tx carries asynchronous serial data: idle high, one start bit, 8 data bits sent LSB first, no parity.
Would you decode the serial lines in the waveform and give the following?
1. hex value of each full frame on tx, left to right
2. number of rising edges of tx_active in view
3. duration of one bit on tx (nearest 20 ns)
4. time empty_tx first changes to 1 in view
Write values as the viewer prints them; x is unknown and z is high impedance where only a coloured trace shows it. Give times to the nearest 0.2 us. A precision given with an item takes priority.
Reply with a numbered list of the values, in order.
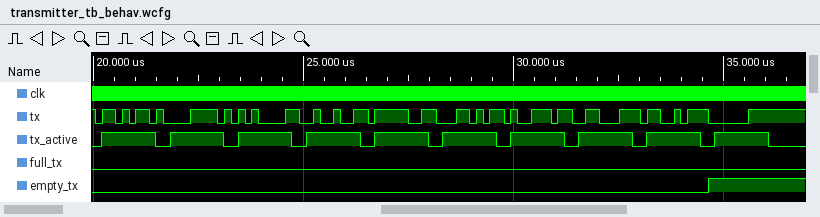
1. 6B, 78, 85, 92, 9F, AC, B9, C6, D3, E0
2. 10
3. 160 ns
4. 34.6 us
